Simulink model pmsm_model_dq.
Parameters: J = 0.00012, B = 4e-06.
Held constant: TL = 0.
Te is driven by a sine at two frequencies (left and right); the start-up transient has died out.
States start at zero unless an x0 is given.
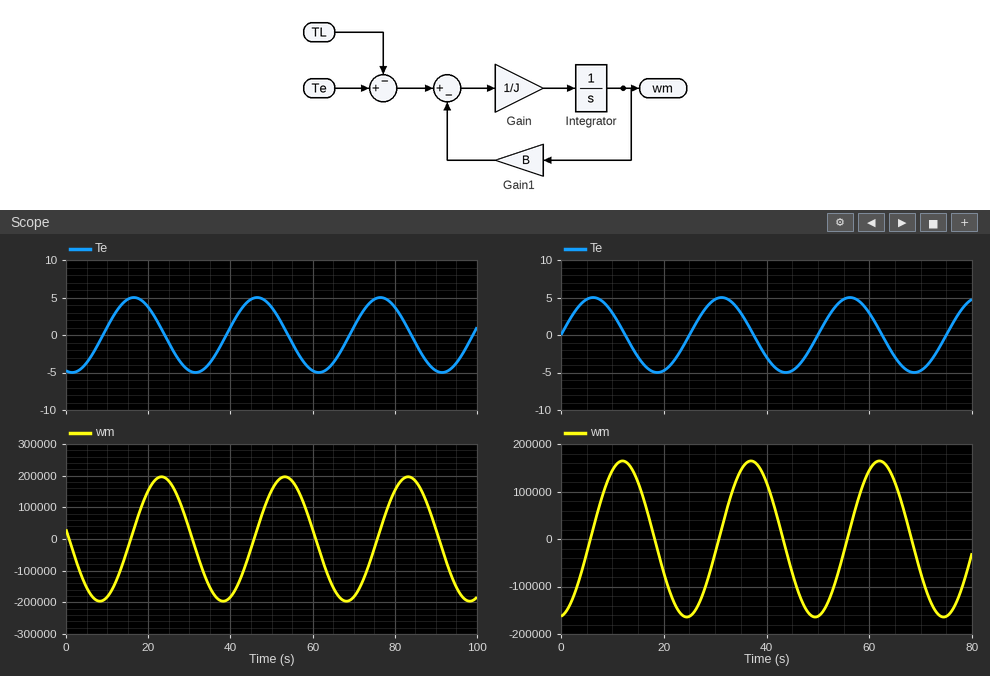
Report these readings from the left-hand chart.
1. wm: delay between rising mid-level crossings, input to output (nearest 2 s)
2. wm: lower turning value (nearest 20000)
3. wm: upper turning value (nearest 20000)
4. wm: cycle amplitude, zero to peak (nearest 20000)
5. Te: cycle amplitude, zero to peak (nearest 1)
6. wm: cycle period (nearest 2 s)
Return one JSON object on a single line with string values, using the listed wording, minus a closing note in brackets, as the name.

{"wm: delay between rising mid-level crossings, input to output": "6 s", "wm: lower turning value": "-200000", "wm: upper turning value": "200000", "wm: cycle amplitude, zero to peak": "200000", "Te: cycle amplitude, zero to peak": "5", "wm: cycle period": "30 s"}
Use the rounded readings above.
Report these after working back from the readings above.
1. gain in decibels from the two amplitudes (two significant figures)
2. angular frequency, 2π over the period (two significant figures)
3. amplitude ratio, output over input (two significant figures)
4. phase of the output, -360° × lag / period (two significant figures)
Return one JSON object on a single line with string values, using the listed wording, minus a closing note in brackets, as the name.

{"gain in decibels from the two amplitudes": "92 dB", "angular frequency, 2π over the period": "0.21 rad/s", "amplitude ratio, output over input": "40000", "phase of the output, -360° × lag / period": "-72°"}
